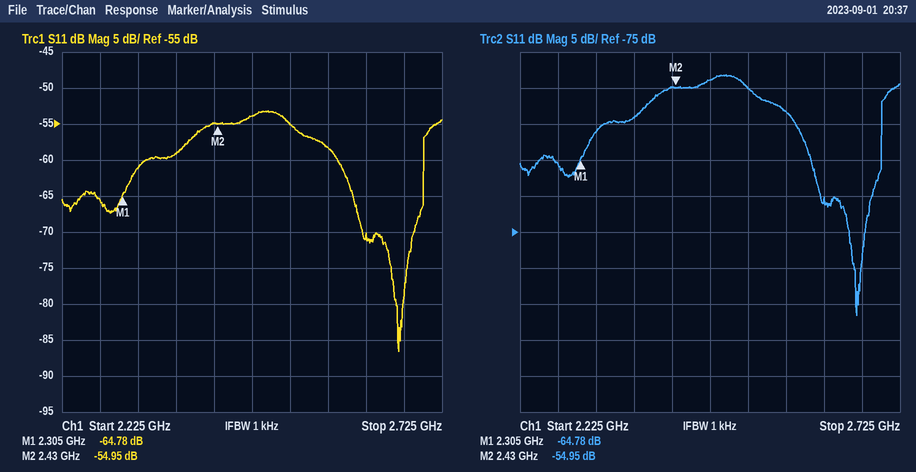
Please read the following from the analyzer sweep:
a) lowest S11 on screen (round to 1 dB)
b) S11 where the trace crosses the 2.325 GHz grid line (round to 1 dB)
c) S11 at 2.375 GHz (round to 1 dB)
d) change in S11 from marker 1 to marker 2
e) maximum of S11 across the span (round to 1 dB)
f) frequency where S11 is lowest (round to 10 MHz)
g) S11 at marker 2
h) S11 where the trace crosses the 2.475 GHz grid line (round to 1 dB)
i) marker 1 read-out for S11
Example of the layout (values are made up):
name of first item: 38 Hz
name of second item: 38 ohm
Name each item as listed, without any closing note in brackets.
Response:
lowest S11 on screen: -87 dB
S11 where the trace crosses the 2.325 GHz grid line: -61 dB
S11 at 2.375 GHz: -59 dB
change in S11 from marker 1 to marker 2: 9.83 dB
maximum of S11 across the span: -53 dB
frequency where S11 is lowest: 2.67 GHz
S11 at marker 2: -54.95 dB
S11 where the trace crosses the 2.475 GHz grid line: -54 dB
marker 1 read-out for S11: -64.78 dB
